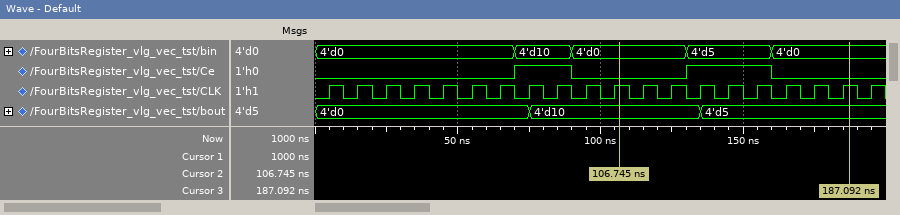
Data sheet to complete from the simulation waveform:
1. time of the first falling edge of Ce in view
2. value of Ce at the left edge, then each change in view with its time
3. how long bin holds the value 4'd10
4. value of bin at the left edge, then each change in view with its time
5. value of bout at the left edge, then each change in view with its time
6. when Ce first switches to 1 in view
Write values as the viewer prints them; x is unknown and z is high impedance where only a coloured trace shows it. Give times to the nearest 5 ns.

90 ns
0, 1 at 70 ns, 0 at 90 ns, 1 at 130 ns, 0 at 160 ns
20 ns
4'd0, 4'd10 at 70 ns, 4'd0 at 90 ns, 4'd5 at 130 ns, 4'd0 at 160 ns
4'd0, 4'd10 at 75 ns, 4'd5 at 135 ns
70 ns
